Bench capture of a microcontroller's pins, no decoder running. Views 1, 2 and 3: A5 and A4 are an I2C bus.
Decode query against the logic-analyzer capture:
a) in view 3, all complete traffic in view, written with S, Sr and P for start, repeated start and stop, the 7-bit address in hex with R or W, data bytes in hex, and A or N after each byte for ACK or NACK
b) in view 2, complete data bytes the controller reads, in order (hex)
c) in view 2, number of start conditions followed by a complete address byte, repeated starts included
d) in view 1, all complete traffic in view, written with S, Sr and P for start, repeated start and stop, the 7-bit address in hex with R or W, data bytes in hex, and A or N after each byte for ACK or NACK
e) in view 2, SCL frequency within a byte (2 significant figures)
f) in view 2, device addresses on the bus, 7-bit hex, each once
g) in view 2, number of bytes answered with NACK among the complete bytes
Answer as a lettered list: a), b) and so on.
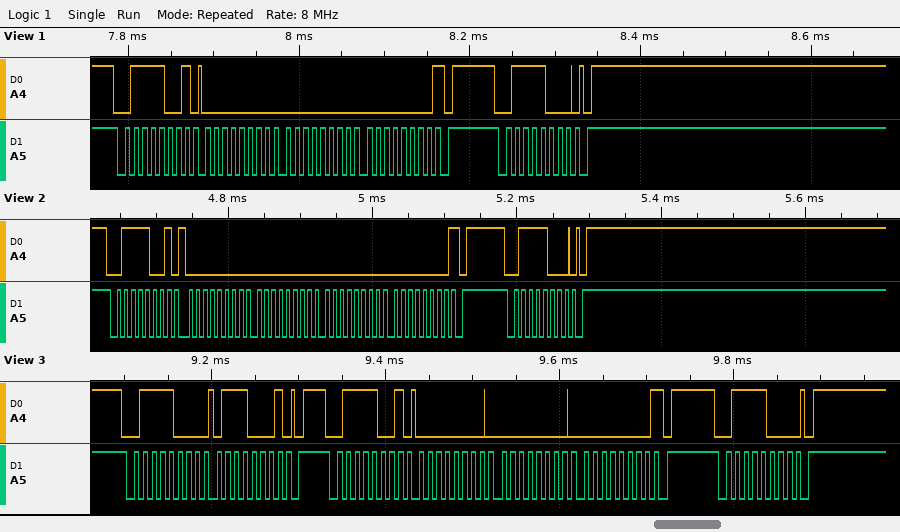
a) S 3CW A 71 A P S 3CR A 00 A 00 A 00 N P S 3CW A P
b) 00 00 00 00
c) 2
d) S 3CR A 00 A 00 A 00 N P S 3CW A P
e) 100 kHz
f) 0x3C
g) 1
